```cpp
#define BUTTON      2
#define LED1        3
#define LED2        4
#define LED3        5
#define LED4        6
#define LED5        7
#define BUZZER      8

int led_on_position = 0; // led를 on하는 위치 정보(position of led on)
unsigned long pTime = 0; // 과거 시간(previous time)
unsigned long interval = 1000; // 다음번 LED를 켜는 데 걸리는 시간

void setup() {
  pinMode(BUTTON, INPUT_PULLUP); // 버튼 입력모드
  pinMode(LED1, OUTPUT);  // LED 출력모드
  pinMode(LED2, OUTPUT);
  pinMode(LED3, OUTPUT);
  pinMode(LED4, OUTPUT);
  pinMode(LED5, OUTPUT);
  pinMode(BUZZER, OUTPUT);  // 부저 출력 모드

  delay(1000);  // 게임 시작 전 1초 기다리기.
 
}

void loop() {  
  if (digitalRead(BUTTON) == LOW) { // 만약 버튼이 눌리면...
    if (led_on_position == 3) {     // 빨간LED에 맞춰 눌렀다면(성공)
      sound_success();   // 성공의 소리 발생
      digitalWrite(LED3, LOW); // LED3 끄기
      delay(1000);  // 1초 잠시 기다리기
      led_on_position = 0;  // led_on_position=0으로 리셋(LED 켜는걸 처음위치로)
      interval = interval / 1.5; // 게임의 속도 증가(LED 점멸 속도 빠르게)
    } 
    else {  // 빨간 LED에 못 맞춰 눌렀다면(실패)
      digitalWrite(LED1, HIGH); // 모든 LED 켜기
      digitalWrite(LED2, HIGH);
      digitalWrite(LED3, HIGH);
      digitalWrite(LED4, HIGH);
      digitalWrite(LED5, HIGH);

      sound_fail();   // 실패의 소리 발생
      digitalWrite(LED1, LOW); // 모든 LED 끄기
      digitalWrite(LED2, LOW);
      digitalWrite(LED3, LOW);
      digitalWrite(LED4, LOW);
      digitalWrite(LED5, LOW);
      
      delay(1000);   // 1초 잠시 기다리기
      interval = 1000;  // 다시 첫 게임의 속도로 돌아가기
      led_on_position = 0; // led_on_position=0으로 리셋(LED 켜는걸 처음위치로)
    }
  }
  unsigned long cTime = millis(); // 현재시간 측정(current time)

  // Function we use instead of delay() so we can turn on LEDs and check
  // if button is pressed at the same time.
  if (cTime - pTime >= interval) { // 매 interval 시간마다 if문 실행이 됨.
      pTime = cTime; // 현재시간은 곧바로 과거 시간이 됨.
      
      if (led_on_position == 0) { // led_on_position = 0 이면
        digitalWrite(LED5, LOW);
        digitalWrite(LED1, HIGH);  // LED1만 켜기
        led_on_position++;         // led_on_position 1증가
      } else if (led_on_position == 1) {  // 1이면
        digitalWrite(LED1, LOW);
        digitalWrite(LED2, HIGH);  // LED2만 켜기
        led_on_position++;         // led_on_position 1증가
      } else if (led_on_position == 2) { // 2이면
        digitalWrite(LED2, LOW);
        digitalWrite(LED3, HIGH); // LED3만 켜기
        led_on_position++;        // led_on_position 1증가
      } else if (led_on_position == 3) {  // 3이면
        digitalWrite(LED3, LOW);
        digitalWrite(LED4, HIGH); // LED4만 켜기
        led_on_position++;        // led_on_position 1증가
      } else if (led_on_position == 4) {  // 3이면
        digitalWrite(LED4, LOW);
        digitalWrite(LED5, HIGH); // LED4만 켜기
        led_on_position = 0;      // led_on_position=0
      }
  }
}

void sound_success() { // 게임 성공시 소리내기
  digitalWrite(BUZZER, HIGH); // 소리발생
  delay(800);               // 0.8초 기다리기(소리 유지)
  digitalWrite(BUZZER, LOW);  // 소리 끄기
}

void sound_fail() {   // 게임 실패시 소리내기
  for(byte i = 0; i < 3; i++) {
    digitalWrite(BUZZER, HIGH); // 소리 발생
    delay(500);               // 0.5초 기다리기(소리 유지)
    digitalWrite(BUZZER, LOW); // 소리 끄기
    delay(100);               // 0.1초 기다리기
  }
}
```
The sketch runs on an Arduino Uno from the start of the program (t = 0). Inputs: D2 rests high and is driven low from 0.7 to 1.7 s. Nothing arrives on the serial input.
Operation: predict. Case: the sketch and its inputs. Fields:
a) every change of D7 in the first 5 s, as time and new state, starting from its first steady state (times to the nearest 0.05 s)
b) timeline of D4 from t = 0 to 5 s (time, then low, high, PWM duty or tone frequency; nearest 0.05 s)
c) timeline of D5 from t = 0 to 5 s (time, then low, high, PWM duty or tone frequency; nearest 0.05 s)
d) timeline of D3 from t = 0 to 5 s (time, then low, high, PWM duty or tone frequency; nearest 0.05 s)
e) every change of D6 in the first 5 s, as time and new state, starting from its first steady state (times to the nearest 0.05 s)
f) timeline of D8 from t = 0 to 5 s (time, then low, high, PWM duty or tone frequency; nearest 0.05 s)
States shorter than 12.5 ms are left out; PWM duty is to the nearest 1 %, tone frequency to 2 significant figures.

0 s low; 1 s high; 2.8 s low
0 s low; 1 s high; 2.8 s low; 4.8 s high
0 s low; 1 s high; 2.8 s low
0 s low; 1 s high; 2.8 s low; 3.8 s high; 4.8 s low
0 s low; 1 s high; 2.8 s low
0 s low; 1 s high; 1.5 s low; 1.6 s high; 2.1 s low; 2.2 s high; 2.7 s low
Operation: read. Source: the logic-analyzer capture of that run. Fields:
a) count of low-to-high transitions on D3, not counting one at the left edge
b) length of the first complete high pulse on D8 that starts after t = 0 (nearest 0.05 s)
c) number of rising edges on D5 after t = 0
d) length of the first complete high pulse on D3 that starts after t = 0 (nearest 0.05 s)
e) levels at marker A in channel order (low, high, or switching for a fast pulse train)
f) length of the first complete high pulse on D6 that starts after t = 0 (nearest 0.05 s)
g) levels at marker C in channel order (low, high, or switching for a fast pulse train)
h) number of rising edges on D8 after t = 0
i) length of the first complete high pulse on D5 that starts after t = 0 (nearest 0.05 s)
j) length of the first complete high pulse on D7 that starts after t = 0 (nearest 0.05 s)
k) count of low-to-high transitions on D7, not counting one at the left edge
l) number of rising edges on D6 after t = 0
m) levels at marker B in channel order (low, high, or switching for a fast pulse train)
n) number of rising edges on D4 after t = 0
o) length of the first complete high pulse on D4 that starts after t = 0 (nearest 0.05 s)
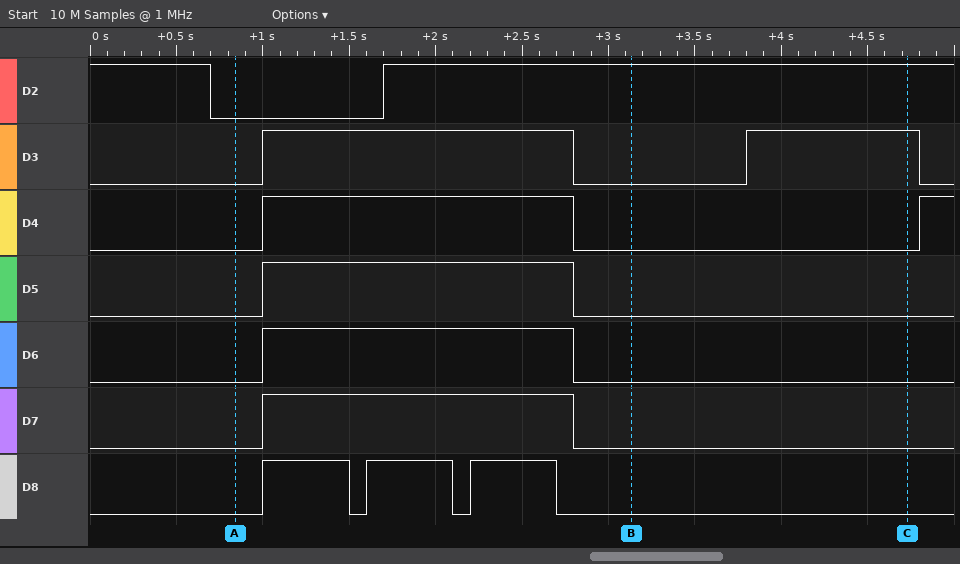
2
0.50 s
1
1.80 s
D2 low, D3 low, D4 low, D5 low, D6 low, D7 low, D8 low
1.80 s
D2 high, D3 high, D4 low, D5 low, D6 low, D7 low, D8 low
3
1.80 s
1.80 s
1
1
D2 high, D3 low, D4 low, D5 low, D6 low, D7 low, D8 low
2
1.80 s
